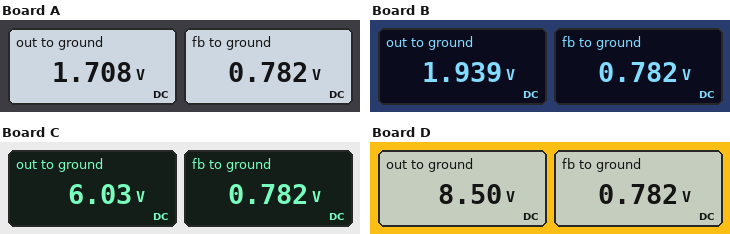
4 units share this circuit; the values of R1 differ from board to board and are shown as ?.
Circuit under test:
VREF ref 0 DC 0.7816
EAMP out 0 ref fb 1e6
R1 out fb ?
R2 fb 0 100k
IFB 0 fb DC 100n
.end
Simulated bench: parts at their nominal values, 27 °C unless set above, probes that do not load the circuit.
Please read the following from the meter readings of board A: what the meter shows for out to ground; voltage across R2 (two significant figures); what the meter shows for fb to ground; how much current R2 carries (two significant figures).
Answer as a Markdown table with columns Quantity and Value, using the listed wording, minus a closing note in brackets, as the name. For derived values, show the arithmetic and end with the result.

| Quantity | Value |
|---|---|
| what the meter shows for out to ground | 1.708 V |
| voltage across R2 | 782 mV = 780 mV |
| what the meter shows for fb to ground | 0.782 V |
| how much current R2 carries | (782 mV) / 100 kΩ = 7.8 µA |
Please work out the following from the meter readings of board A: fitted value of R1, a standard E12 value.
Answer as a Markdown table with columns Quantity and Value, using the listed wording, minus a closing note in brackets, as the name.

| Quantity | Value |
|---|---|
| fitted value of R1, a standard E12 value | 120 kΩ |
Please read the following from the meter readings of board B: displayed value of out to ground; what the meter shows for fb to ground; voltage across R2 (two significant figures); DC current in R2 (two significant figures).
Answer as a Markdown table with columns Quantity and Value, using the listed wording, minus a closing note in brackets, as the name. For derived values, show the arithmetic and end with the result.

| Quantity | Value |
|---|---|
| displayed value of out to ground | 1.939 V |
| what the meter shows for fb to ground | 0.782 V |
| voltage across R2 | 782 mV = 780 mV |
| DC current in R2 | (782 mV) / 100 kΩ = 7.8 µA |
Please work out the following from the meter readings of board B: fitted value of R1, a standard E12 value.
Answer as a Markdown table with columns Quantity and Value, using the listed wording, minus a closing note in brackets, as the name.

| Quantity | Value |
|---|---|
| fitted value of R1, a standard E12 value | 150 kΩ |
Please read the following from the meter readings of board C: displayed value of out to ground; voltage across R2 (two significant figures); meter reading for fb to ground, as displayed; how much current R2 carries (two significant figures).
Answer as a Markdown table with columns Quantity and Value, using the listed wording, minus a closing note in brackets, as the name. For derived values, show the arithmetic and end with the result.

| Quantity | Value |
|---|---|
| displayed value of out to ground | 6.03 V |
| voltage across R2 | 782 mV = 780 mV |
| meter reading for fb to ground, as displayed | 0.782 V |
| how much current R2 carries | (782 mV) / 100 kΩ = 7.8 µA |
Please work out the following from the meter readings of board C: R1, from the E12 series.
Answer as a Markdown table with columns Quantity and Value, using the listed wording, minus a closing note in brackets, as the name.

| Quantity | Value |
|---|---|
| R1, from the E12 series | 680 kΩ |
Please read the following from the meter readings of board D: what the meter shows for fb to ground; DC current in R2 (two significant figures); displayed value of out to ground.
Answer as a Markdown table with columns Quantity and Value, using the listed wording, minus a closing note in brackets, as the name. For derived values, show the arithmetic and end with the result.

| Quantity | Value |
|---|---|
| what the meter shows for fb to ground | 0.782 V |
| DC current in R2 | (782 mV) / 100 kΩ = 7.8 µA |
| displayed value of out to ground | 8.50 V |
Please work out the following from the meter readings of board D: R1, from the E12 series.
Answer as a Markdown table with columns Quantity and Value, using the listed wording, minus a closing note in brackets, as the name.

| Quantity | Value |
|---|---|
| R1, from the E12 series | 1 MΩ |
